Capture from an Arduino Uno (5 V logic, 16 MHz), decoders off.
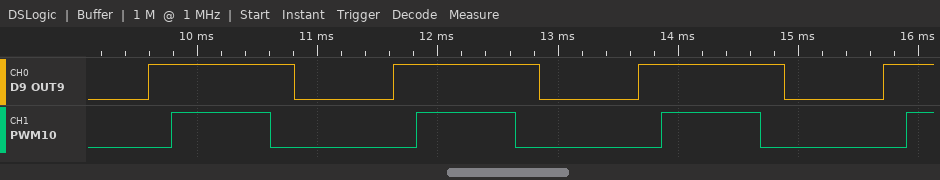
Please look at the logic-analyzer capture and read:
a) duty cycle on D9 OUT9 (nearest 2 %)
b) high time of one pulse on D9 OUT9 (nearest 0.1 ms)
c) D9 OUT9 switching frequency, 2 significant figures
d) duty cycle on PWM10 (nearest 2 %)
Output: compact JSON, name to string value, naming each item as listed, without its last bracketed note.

{"duty cycle on D9 OUT9": "60 %", "high time of one pulse on D9 OUT9": "1.2 ms", "D9 OUT9 switching frequency, 2 significant figures": "490 Hz", "duty cycle on PWM10": "40 %"}
